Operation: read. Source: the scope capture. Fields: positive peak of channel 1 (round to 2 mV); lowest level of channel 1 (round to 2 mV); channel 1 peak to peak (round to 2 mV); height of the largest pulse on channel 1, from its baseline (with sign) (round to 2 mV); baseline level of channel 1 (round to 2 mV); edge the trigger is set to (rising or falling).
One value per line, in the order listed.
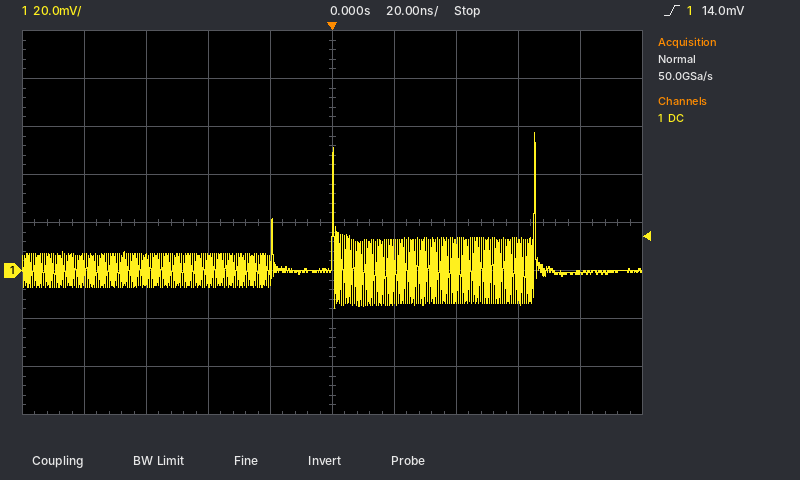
58 mV
-16 mV
74 mV
+58 mV
0 mV
rising
